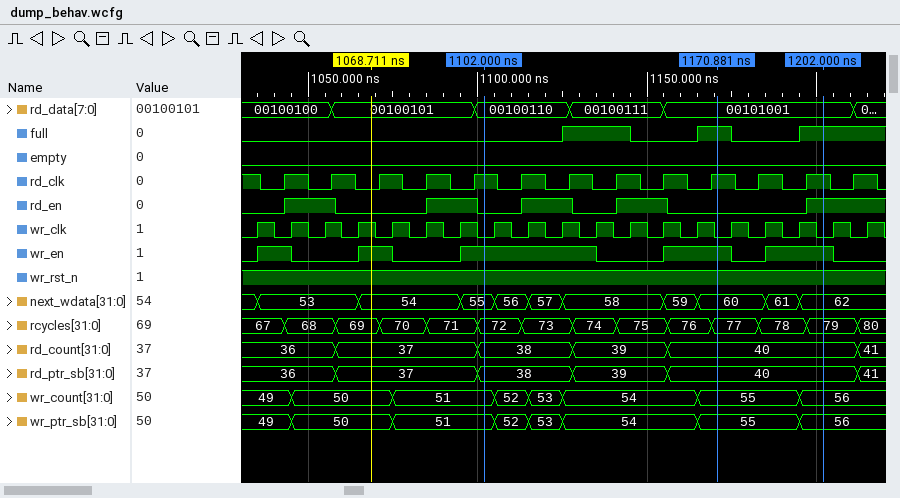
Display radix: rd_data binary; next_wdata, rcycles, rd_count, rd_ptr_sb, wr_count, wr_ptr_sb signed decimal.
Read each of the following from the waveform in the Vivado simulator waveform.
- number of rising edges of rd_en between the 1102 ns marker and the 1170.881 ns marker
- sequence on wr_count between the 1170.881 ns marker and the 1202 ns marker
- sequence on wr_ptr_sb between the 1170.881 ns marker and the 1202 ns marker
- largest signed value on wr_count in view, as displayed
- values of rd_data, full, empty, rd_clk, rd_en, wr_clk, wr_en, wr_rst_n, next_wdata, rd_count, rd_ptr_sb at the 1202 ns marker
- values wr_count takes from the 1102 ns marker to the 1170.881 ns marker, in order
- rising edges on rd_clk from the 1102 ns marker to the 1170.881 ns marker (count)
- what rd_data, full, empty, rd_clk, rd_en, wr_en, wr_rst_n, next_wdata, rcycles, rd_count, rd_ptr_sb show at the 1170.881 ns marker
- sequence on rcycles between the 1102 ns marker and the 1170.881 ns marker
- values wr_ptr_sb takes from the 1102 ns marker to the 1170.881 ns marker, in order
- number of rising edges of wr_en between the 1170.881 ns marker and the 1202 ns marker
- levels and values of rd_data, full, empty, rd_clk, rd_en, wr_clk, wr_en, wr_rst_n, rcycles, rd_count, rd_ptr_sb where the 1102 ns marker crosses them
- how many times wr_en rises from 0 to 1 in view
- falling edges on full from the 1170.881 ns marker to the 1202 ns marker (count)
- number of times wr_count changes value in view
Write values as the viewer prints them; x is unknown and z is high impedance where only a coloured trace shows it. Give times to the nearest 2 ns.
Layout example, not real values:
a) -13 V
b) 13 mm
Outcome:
a) 2
b) 55, 56
c) 55, 56
d) 56
e) rd_data=00101001, full=1, empty=0, rd_clk=1, rd_en=1, wr_clk=0, wr_en=1, wr_rst_n=1, next_wdata=62, rd_count=40, rd_ptr_sb=40
f) 51, 52, 53, 54, 55
g) 5
h) rd_data=00101001, full=1, empty=0, rd_clk=1, rd_en=0, wr_en=1, wr_rst_n=1, next_wdata=60, rcycles=77, rd_count=40, rd_ptr_sb=40
i) 72, 73, 74, 75, 76, 77
j) 51, 52, 53, 54, 55
k) 1
l) rd_data=00100110, full=0, empty=0, rd_clk=1, rd_en=0, wr_clk=0, wr_en=1, wr_rst_n=1, rcycles=72, rd_count=38, rd_ptr_sb=38
m) 5
n) 1
o) 7
